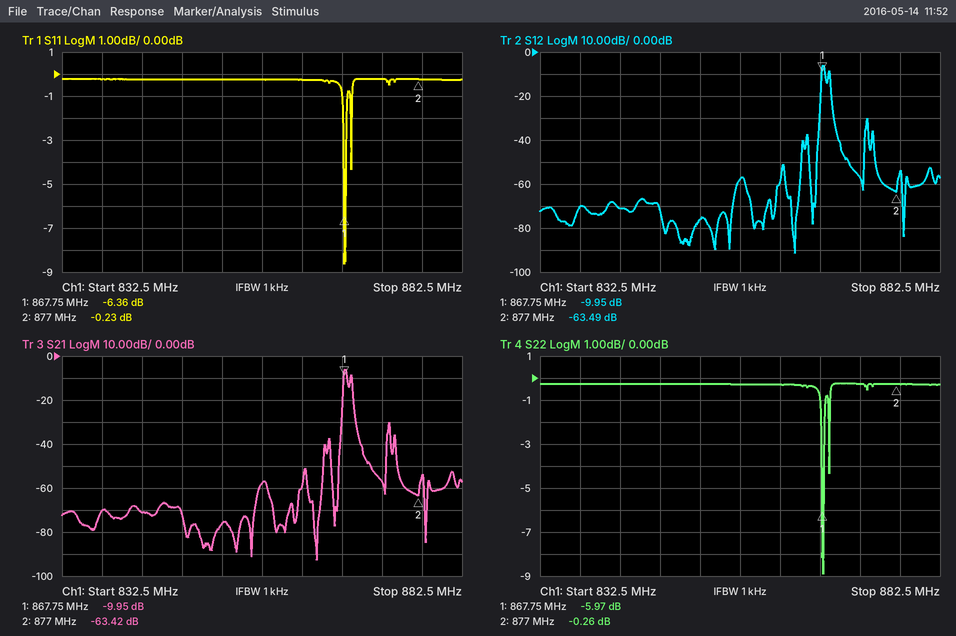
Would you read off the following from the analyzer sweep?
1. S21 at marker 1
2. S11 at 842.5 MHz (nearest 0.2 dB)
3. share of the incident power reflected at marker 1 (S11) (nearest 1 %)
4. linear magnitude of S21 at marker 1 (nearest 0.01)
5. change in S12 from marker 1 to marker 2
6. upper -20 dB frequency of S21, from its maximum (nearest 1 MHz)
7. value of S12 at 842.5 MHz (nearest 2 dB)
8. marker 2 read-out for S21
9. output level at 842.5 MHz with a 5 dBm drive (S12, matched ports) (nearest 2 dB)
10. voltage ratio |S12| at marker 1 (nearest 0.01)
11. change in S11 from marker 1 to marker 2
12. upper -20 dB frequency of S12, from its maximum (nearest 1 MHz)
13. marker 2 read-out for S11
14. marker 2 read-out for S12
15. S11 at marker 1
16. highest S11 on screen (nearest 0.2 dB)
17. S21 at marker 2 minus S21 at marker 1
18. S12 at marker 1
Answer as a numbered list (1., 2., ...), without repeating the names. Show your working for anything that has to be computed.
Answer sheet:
1. -9.95 dB
2. -0.2 dB
3. 10^(-6.36/10) ≈ 23 %
4. 10^(-9.95/20) ≈ 0.32
5. -63.49 − (-9.95) = -53.54 dB
6. 869 MHz
7. -72 dB
8. -63.42 dB
9. 5 dBm + (-72 dB) = -66 dBm
10. 10^(-9.95/20) ≈ 0.32
11. -0.23 − (-6.36) = 6.13 dB
12. 869 MHz
13. -0.23 dB
14. -63.49 dB
15. -6.36 dB
16. -0.2 dB
17. -63.42 − (-9.95) = -53.47 dB
18. -9.95 dB
